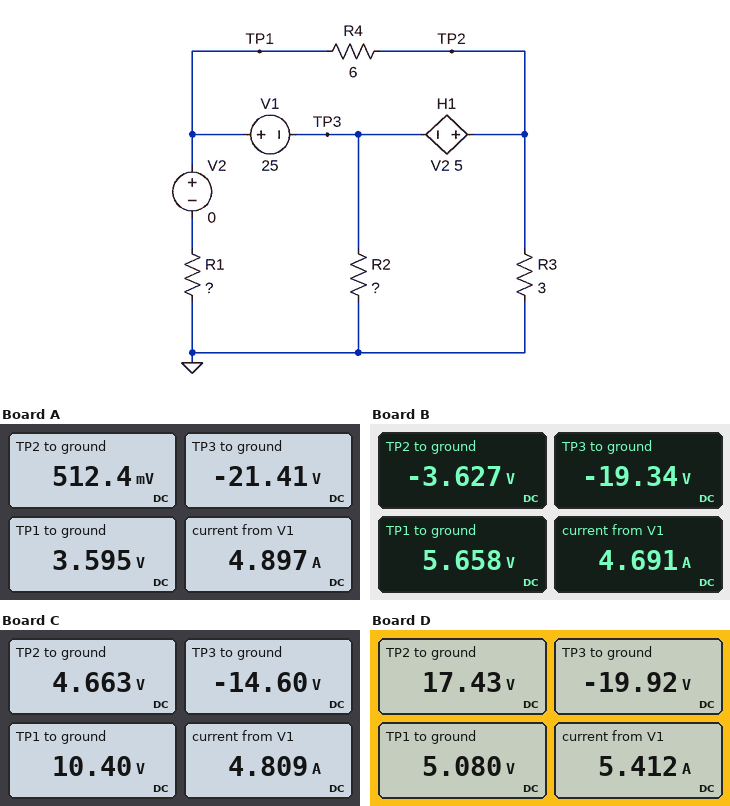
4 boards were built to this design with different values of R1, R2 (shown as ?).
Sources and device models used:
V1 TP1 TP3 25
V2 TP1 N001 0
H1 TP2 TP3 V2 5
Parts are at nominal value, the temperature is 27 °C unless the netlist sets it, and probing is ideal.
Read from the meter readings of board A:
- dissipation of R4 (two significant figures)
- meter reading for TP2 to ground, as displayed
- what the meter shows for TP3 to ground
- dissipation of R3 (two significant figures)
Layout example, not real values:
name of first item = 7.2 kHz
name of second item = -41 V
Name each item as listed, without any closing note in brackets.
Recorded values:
dissipation of R4 = 1.6 W
meter reading for TP2 to ground, as displayed = 512.4 mV
what the meter shows for TP3 to ground = -21.41 V
dissipation of R3 = 88 mW
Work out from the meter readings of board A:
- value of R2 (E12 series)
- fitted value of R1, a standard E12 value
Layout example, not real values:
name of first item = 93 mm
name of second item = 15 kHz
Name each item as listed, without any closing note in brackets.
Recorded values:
value of R2 = 4.7 Ω
fitted value of R1, a standard E12 value = 0.82 Ω
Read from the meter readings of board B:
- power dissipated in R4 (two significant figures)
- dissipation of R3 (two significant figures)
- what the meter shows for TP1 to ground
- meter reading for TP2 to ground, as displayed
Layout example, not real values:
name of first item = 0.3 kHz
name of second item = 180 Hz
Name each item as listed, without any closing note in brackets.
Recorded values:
power dissipated in R4 = 14 W
dissipation of R3 = 4.4 W
what the meter shows for TP1 to ground = 5.658 V
meter reading for TP2 to ground, as displayed = -3.627 V
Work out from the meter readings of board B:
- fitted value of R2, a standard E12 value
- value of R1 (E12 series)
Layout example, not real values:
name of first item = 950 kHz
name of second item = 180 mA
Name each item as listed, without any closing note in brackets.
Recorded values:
fitted value of R2, a standard E12 value = 10 Ω
value of R1 = 1.8 Ω
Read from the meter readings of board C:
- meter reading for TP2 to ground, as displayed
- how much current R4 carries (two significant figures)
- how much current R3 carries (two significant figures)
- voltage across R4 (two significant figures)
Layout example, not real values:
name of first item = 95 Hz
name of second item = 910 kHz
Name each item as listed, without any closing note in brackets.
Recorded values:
meter reading for TP2 to ground, as displayed = 4.663 V
how much current R4 carries = 960 mA
how much current R3 carries = 1.6 A
voltage across R4 = 5.7 V
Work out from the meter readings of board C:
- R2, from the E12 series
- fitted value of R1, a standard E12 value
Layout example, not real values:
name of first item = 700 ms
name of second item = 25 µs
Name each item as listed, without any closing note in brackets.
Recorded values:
R2, from the E12 series = 2.7 Ω
fitted value of R1, a standard E12 value = 2.7 Ω
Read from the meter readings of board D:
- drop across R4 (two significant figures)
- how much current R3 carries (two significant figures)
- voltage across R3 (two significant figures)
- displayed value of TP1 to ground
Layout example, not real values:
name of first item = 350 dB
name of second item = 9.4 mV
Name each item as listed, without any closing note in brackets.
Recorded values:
drop across R4 = 12 V
how much current R3 carries = 5.8 A
voltage across R3 = 17 V
displayed value of TP1 to ground = 5.080 V
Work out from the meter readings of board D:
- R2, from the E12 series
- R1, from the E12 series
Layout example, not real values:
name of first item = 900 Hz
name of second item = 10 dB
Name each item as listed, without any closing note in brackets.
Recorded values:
R2, from the E12 series = 1.5 Ω
R1, from the E12 series = 0.68 Ω
